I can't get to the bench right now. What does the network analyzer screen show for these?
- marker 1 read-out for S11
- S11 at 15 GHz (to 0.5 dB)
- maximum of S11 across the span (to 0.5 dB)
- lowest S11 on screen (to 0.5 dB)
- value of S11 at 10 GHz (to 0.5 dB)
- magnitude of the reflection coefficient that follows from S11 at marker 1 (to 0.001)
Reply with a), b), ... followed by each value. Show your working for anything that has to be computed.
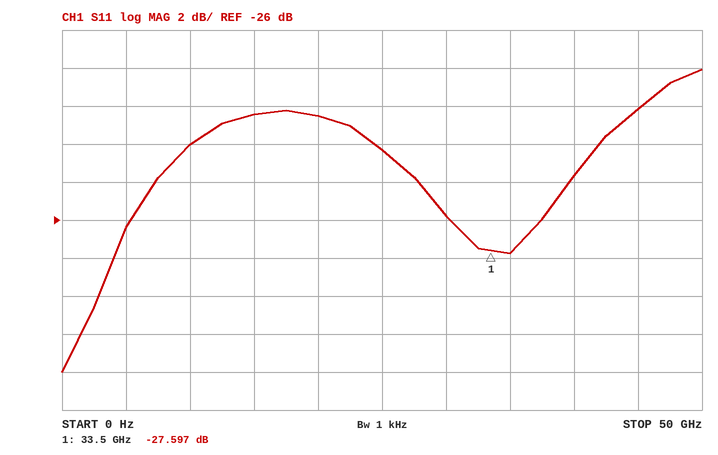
a) -27.597 dB
b) -20.5 dB
c) -18.0 dB
d) -34.0 dB
e) -22.0 dB
f) 10^(-27.597/20) ≈ 0.042
